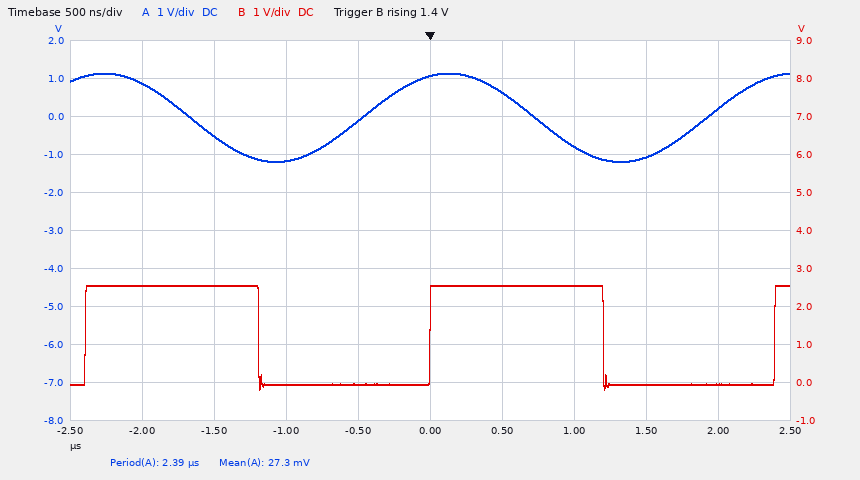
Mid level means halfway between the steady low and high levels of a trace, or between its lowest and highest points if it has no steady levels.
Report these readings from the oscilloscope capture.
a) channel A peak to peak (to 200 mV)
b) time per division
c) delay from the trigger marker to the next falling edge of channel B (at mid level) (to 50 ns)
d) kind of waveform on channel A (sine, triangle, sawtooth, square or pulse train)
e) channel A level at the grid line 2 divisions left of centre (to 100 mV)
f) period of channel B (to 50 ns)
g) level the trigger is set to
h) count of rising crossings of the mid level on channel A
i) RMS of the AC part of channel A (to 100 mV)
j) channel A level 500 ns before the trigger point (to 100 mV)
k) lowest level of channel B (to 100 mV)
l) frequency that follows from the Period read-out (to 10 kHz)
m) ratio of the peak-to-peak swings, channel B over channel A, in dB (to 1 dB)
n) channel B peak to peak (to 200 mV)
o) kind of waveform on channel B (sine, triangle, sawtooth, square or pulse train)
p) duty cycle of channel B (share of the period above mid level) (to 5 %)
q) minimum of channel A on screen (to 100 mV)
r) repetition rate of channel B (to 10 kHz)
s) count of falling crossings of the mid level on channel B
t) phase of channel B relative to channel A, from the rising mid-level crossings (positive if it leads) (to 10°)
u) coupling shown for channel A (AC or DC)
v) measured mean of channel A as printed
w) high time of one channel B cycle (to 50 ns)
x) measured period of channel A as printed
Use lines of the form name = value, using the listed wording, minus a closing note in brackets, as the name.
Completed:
channel A peak to peak = 2.4 V
time per division = 500 ns
delay from the trigger marker to the next falling edge of channel B (at mid level) = 1.20 µs
kind of waveform on channel A = sine
channel A level at the grid line 2 divisions left of centre = -1.2 V
period of channel B = 2.40 µs
level the trigger is set to = 1.4 V
count of rising crossings of the mid level on channel A = 2
RMS of the AC part of channel A = 800 mV
channel A level 500 ns before the trigger point = -100 mV
lowest level of channel B = -200 mV
frequency that follows from the Period read-out = 420 kHz
ratio of the peak-to-peak swings, channel B over channel A, in dB = 1 dB
channel B peak to peak = 2.8 V
kind of waveform on channel B = square
duty cycle of channel B (share of the period above mid level) = 50 %
minimum of channel A on screen = -1.2 V
repetition rate of channel B = 420 kHz
count of falling crossings of the mid level on channel B = 2
phase of channel B relative to channel A, from the rising mid-level crossings (positive if it leads) = -70°
coupling shown for channel A = DC
measured mean of channel A as printed = 27.3 mV
high time of one channel B cycle = 1.20 µs
measured period of channel A as printed = 2.39 µs
